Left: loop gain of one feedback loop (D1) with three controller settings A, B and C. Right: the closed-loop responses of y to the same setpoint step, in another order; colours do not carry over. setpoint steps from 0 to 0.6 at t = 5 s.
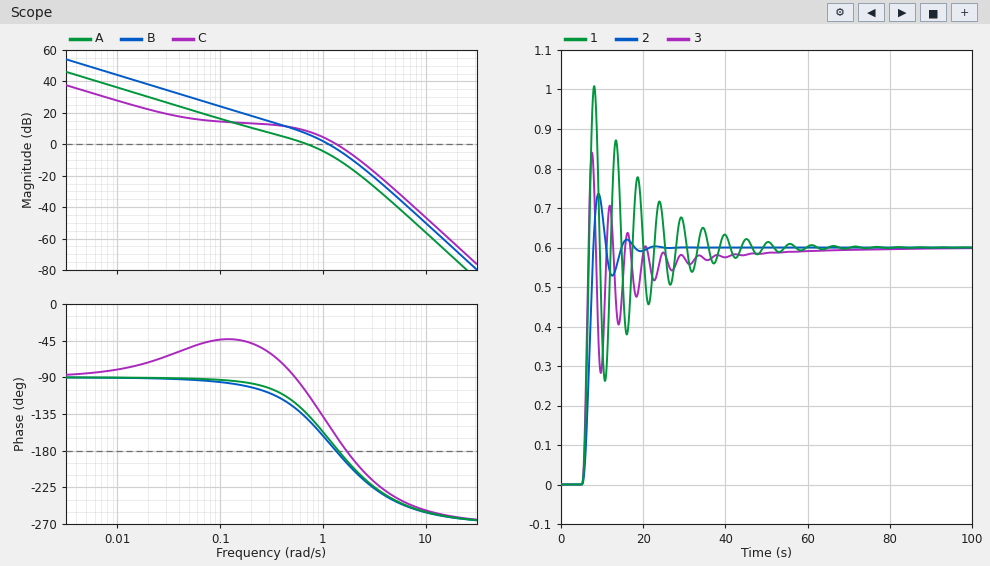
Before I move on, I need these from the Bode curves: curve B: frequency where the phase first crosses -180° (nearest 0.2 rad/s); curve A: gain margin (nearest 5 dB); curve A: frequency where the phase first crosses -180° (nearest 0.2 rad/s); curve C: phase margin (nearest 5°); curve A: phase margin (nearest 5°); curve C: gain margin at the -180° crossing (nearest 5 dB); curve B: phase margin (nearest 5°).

1.4 rad/s
10 dB
1.4 rad/s
15°
45°
5 dB
10°
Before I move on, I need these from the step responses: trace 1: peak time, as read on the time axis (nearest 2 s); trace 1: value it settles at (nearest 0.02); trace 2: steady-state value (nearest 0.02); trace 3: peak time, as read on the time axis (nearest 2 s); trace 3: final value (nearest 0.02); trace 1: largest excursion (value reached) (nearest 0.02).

8 s
0.60
0.60
8 s
0.60
1.00
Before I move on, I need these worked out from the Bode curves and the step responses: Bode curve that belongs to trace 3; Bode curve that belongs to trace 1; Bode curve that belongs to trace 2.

C
B
A
